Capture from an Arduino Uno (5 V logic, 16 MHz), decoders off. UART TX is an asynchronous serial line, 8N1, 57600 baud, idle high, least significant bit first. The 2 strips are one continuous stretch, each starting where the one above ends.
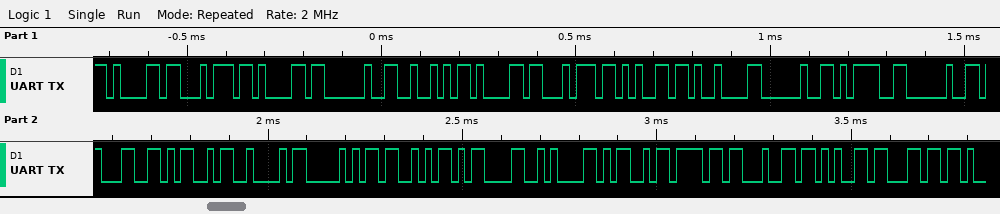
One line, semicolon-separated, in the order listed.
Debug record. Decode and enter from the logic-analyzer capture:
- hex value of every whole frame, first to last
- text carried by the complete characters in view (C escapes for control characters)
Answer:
0x61 0x74 0x61 0x20 0x52 0x61 0x74 0x65 0x09 0x20 0x3D 0x20 0x31 0x4D 0x42 0x50 0x53 0x0D 0x0A 0x4D 0x6F 0x64 0x65 0x6C; "ata Rate\t = 1MBPS\r\nModel"
